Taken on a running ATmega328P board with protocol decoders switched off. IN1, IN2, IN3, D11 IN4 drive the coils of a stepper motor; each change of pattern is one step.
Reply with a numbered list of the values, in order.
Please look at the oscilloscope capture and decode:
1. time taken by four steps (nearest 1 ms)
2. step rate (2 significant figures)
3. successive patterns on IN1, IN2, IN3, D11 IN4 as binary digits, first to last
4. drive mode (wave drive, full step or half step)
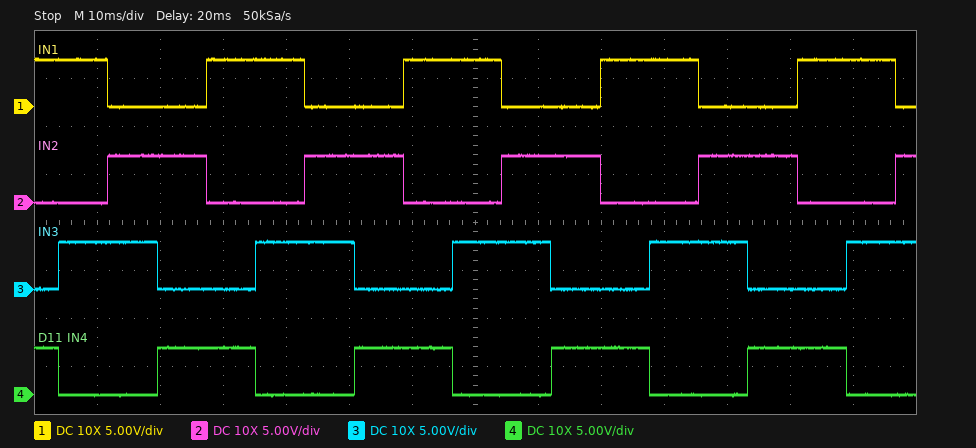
1. 31 ms
2. 130 steps/s
3. 1001 1010 0110 0101 1001 1010 0110 0101 1001 1010 0110 0101 1001 1010 0110 0101 1001 1010 0110
4. full step
